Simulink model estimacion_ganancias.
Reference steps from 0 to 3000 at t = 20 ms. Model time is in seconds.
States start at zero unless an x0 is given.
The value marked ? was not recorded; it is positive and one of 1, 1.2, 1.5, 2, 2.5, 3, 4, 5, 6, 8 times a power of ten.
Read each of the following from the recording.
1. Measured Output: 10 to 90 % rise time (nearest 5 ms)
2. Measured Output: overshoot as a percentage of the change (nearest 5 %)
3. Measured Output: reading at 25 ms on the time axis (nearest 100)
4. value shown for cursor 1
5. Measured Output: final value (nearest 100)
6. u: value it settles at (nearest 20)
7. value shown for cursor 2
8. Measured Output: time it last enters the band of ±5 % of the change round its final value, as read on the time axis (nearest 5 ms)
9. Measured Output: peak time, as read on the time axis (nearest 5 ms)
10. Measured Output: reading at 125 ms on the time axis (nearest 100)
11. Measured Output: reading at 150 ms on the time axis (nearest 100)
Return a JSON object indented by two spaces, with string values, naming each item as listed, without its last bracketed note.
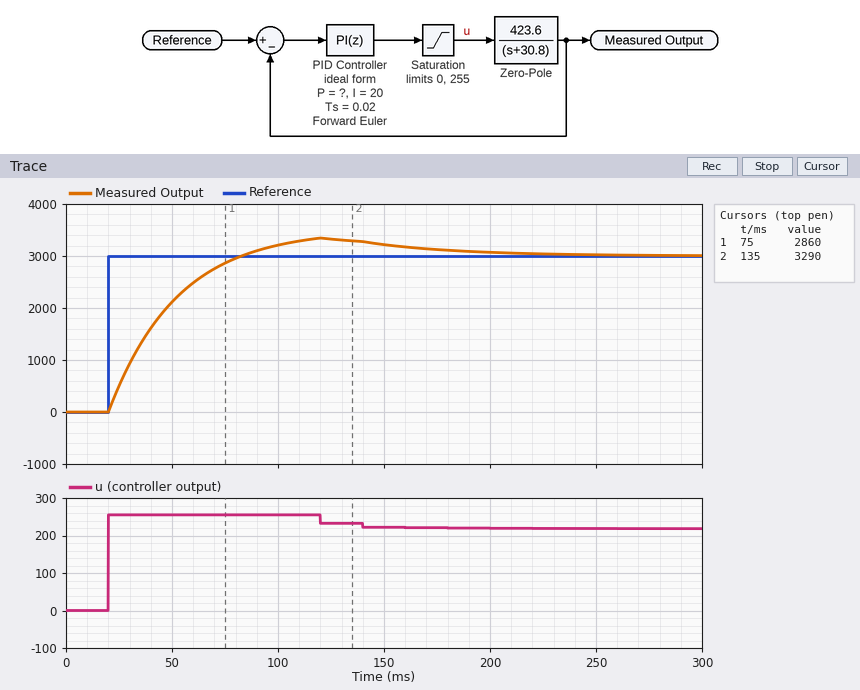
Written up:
{
  "Measured Output: 10 to 90 % rise time": "45 ms",
  "Measured Output: overshoot as a percentage of the change": "10 %",
  "Measured Output: reading at 25 ms on the time axis": "500",
  "value shown for cursor 1": "2860",
  "Measured Output: final value": "3000",
  "u: value it settles at": "220",
  "value shown for cursor 2": "3290",
  "Measured Output: time it last enters the band of ±5 % of the change round its final value, as read on the time axis": "165 ms",
  "Measured Output: peak time, as read on the time axis": "120 ms",
  "Measured Output: reading at 125 ms on the time axis": "3300",
  "Measured Output: reading at 150 ms on the time axis": "3200"
}
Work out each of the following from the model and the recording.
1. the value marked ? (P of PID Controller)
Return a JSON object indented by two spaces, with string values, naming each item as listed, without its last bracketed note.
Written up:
{
  "the value marked ?": "0.15"
}
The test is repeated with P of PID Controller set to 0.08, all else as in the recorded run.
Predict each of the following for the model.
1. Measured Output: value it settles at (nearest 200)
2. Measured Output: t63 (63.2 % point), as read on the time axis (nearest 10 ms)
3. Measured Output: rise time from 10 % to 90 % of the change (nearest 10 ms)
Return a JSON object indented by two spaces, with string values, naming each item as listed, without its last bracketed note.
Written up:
{
  "Measured Output: value it settles at": "3000",
  "Measured Output: t63 (63.2 % point), as read on the time axis": "50 ms",
  "Measured Output: rise time from 10 % to 90 % of the change": "80 ms"
}
